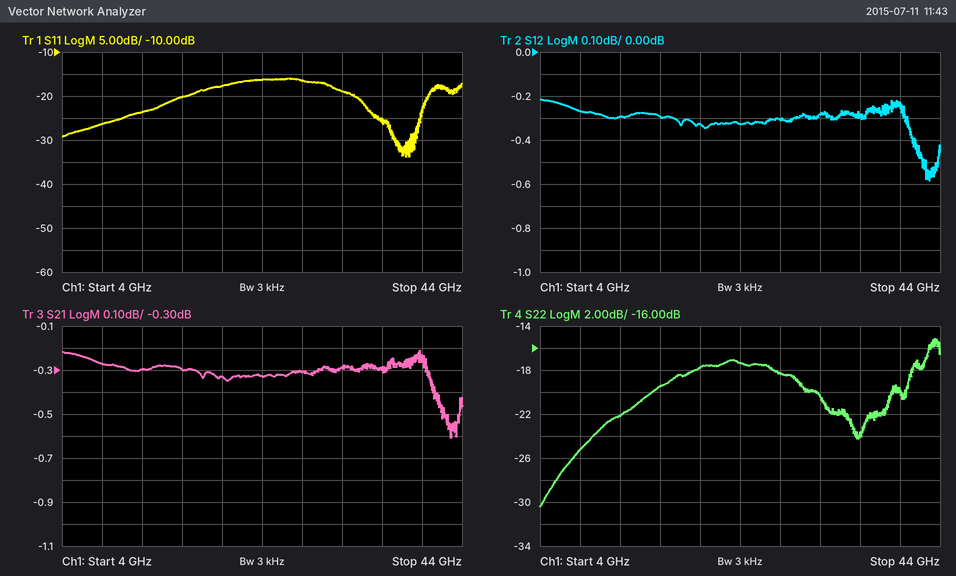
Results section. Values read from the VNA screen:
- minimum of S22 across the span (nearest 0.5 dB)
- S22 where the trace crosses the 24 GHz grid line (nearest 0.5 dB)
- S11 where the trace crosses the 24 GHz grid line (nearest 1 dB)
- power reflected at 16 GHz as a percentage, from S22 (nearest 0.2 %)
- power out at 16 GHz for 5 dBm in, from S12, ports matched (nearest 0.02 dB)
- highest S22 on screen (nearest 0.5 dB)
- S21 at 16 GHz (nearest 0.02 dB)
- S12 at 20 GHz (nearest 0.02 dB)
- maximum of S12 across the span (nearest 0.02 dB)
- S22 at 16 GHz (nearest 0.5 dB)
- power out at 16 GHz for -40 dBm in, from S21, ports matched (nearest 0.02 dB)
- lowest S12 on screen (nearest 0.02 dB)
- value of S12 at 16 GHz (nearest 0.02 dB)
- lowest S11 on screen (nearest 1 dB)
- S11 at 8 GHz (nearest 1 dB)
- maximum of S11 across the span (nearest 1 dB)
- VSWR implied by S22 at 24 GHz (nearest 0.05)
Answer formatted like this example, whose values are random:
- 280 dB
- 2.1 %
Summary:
- -30.5 dB
- -17.5 dB
- -16 dB
- 1.2 %
- 4.70 dBm
- -15.0 dB
- -0.30 dB
- -0.32 dB
- -0.22 dB
- -19.5 dB
- -40.30 dBm
- -0.58 dB
- -0.30 dB
- -34 dB
- -26 dB
- -16 dB
- 1.30
